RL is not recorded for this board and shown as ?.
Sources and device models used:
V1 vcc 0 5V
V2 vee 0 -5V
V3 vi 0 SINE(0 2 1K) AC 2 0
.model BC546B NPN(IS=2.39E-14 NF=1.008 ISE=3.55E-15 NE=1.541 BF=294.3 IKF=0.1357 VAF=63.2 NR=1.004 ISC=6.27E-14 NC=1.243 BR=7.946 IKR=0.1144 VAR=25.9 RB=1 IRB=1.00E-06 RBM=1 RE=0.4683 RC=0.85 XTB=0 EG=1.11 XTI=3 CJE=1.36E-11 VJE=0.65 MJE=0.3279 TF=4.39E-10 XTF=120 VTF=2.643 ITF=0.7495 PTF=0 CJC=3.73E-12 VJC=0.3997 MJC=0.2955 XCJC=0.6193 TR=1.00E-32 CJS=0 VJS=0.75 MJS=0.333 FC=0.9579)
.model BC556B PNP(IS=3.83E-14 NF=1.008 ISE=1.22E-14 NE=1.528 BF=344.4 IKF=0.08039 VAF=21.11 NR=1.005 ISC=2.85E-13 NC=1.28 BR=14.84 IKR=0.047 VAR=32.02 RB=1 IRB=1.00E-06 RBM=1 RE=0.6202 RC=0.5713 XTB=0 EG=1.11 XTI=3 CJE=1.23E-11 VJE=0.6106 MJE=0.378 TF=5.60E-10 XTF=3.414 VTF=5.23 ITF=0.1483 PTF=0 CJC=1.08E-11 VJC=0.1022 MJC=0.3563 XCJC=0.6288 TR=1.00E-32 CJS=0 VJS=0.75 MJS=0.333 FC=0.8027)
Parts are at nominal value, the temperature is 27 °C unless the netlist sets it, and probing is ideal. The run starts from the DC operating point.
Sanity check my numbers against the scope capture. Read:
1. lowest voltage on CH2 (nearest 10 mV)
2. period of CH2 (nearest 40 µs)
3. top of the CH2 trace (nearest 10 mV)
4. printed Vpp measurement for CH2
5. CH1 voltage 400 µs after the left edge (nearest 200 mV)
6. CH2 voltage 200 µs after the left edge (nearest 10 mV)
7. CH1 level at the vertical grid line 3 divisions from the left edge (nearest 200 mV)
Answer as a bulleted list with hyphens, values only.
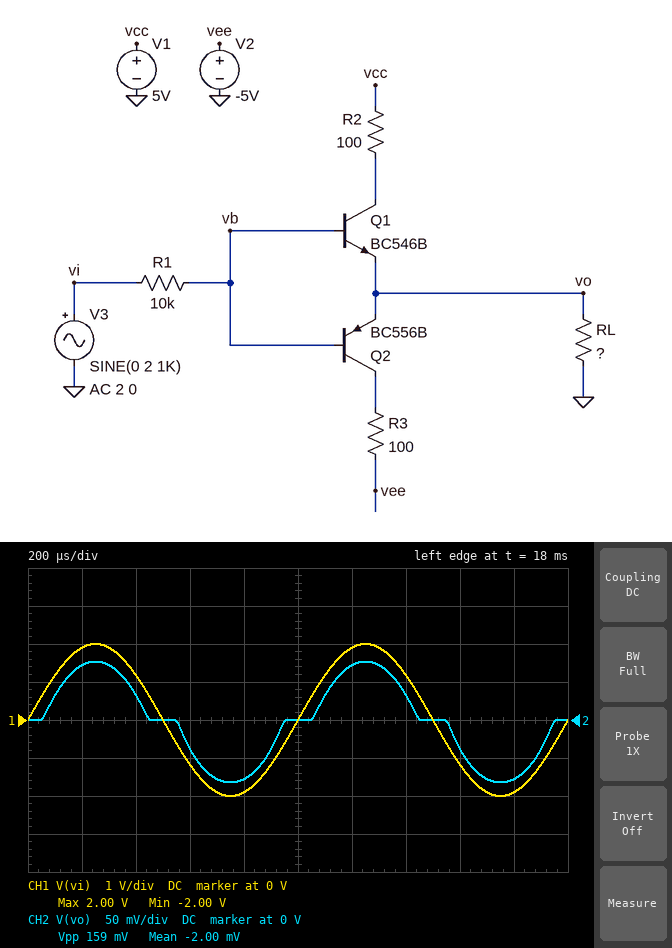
- -80 mV
- 1.00 ms
- 80 mV
- 159 mV
- 1.2 V
- 70 mV
- -1.2 V
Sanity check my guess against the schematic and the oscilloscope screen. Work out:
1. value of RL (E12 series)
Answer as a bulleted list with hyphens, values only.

- 2.7 Ω
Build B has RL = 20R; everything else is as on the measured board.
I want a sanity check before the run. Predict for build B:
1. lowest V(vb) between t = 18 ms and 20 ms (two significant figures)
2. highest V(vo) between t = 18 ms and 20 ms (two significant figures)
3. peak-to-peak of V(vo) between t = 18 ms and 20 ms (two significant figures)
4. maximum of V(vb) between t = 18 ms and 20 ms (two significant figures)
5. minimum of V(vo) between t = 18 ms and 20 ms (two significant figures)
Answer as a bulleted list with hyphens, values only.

- -1.2 V
- 430 mV
- 890 mV
- 1.2 V
- -460 mV
